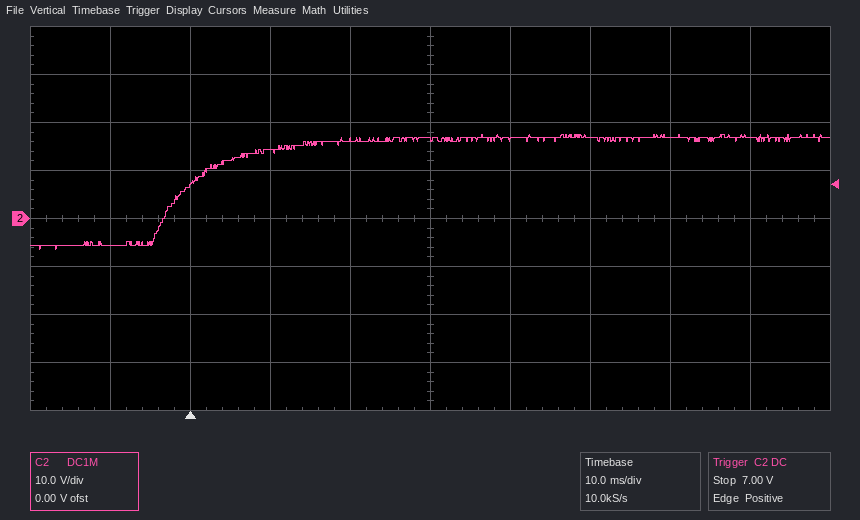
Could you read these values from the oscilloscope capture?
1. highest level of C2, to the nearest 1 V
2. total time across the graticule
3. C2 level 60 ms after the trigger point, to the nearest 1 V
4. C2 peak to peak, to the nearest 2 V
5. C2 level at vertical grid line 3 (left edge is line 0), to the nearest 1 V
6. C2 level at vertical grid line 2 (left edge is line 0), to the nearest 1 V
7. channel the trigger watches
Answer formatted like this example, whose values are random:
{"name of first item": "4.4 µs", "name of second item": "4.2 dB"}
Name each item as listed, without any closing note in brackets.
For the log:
{"highest level of C2, to the nearest 1 V": "18 V", "total time across the graticule": "100 ms", "C2 level 60 ms after the trigger point, to the nearest 1 V": "17 V", "C2 peak to peak, to the nearest 2 V": "24 V", "C2 level at vertical grid line 3 (left edge is line 0), to the nearest 1 V": "14 V", "C2 level at vertical grid line 2 (left edge is line 0), to the nearest 1 V": "7 V", "channel the trigger watches": "C2"}
